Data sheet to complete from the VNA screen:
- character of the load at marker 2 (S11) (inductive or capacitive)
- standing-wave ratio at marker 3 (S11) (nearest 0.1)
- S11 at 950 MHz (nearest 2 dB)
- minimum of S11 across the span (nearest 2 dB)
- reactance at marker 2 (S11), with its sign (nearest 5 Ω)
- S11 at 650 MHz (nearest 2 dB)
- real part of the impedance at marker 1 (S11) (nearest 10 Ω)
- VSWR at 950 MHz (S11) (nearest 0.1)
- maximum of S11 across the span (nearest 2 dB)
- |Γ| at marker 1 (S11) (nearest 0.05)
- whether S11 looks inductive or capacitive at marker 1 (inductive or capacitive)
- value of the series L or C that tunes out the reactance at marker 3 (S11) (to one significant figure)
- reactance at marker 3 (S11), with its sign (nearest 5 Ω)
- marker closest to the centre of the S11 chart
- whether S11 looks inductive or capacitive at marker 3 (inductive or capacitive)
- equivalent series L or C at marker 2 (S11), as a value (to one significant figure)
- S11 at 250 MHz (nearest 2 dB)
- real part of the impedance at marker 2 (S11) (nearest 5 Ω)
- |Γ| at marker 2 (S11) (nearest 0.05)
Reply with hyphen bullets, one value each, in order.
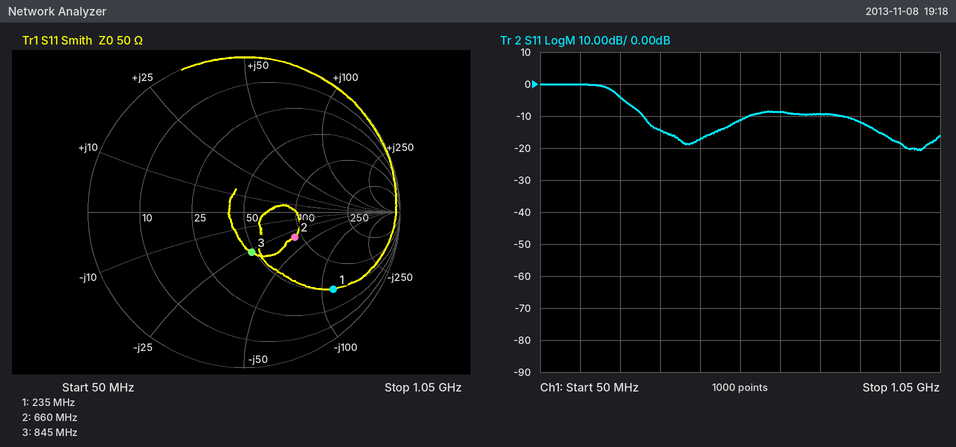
- capacitive
- 1.7
- -18 dB
- -20 dB
- -35 Ω
- -8 dB
- 50 Ω
- 1.3
- 0 dB
- 0.75
- capacitive
- 5 nH
- -25 Ω
- marker 3
- capacitive
- 7 pF
- -4 dB
- 90 Ω
- 0.35
